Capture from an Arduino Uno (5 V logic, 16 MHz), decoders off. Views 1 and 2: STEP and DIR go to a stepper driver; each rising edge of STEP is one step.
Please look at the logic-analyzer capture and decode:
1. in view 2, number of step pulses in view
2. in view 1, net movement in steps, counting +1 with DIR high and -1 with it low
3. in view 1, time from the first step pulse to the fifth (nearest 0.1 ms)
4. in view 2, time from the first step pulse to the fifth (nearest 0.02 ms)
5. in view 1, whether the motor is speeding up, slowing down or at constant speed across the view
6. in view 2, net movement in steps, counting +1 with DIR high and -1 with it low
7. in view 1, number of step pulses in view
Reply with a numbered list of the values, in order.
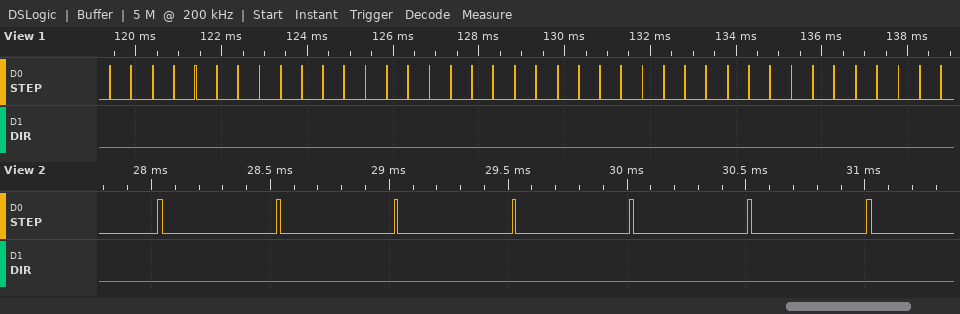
1. 7
2. -40
3. 2.0 ms
4. 1.98 ms
5. constant speed
6. -7
7. 40
